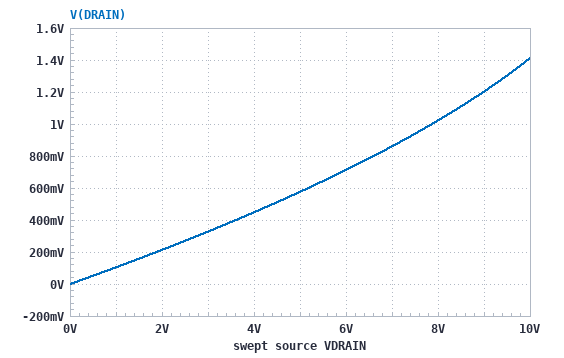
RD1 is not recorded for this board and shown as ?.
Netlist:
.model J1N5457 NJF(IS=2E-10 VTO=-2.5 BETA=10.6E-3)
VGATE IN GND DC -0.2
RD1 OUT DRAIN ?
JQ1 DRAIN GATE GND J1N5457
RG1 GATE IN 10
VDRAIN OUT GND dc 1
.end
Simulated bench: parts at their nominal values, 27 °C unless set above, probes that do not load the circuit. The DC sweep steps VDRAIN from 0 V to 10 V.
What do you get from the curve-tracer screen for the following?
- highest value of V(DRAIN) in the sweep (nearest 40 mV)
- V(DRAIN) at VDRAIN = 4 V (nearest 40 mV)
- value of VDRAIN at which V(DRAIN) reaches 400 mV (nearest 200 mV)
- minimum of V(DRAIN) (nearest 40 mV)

1.40 V
440 mV
3.6 V
0 V
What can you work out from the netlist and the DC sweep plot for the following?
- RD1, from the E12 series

180 Ω
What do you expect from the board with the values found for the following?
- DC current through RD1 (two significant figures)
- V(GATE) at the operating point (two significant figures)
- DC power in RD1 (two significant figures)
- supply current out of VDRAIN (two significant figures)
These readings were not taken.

5.0 mA
-200 mV
4.5 mW
5.0 mA
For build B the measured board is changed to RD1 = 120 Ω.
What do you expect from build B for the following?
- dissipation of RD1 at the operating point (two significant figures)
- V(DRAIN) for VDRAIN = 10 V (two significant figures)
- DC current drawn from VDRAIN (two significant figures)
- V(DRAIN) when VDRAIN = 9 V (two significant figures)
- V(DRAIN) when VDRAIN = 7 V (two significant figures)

6.0 mW
3.3 V
7.1 mA
2.3 V
1.4 V
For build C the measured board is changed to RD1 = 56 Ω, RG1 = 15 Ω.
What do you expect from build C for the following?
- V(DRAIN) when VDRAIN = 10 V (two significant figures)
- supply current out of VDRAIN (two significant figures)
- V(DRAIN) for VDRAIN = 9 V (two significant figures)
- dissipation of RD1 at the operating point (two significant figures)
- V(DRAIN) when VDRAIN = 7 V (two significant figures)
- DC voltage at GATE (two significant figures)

6.9 V
13 mA
5.9 V
9.2 mW
3.9 V
-200 mV
